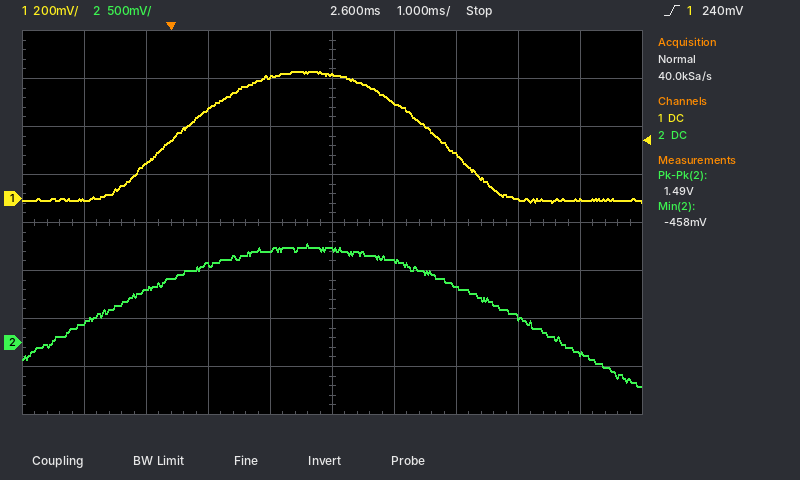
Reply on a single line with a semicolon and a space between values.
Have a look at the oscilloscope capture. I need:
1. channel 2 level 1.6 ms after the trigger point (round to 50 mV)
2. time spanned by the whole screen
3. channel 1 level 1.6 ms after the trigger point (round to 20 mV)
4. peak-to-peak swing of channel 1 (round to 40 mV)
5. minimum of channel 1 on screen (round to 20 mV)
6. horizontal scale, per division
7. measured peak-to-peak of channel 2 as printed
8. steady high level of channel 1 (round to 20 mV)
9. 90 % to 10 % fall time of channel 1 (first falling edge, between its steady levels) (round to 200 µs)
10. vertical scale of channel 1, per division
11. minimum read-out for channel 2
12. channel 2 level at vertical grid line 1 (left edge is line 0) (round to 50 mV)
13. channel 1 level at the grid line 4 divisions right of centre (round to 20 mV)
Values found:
950 mV; 10 ms; 500 mV; 560 mV; -20 mV; 1 ms; 1.49 V; 520 mV; 2.0 ms; 200 mV; -458 mV; 200 mV; 0 mV
